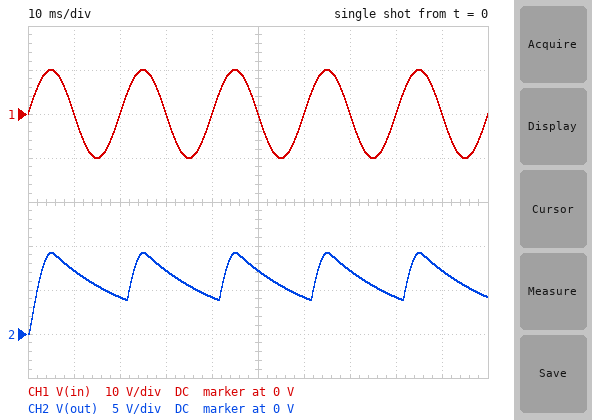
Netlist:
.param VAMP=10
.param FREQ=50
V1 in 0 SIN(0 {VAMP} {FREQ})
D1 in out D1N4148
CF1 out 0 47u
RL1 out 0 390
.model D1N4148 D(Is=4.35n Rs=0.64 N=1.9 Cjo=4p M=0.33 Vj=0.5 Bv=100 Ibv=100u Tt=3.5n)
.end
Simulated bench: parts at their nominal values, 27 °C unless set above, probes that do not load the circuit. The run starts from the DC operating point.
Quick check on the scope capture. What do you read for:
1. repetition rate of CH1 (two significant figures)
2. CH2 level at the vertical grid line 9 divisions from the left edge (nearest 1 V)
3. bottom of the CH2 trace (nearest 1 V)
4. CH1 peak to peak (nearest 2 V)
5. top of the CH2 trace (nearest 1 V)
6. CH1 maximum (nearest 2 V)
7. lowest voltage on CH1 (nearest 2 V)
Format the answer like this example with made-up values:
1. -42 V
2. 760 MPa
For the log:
1. 50 Hz
2. 7 V
3. 0 V
4. 20 V
5. 9 V
6. 10 V
7. -10 V
